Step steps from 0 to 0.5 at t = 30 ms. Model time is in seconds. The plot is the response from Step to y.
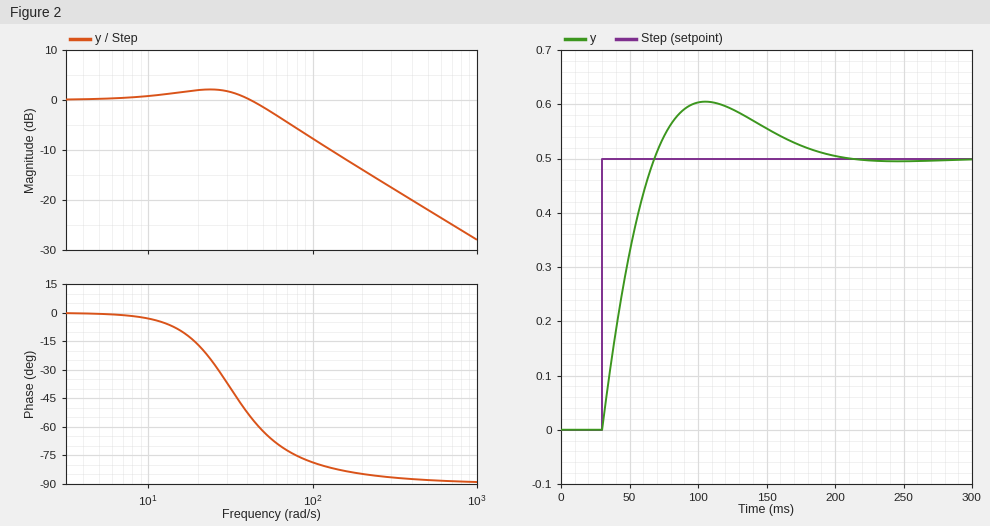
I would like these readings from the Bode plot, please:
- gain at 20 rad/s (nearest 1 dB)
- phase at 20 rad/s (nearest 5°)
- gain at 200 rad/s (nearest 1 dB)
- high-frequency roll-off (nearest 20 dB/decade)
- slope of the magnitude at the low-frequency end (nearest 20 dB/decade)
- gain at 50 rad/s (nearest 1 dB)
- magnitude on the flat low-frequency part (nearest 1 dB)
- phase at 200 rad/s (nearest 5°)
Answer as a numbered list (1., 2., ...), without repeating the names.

1. 2 dB
2. -15°
3. -14 dB
4. -20 dB/decade
5. 0 dB/decade
6. -1 dB
7. 0 dB
8. -85°
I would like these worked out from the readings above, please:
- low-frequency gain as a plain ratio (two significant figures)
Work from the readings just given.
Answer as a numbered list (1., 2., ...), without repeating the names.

1. 1.0
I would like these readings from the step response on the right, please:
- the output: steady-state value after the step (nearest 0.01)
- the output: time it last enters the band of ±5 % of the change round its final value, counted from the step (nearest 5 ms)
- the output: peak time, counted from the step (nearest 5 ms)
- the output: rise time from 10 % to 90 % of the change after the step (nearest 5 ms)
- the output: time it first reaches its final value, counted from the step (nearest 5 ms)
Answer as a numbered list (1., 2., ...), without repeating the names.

1. 0.50
2. 145 ms
3. 75 ms
4. 30 ms
5. 40 ms
